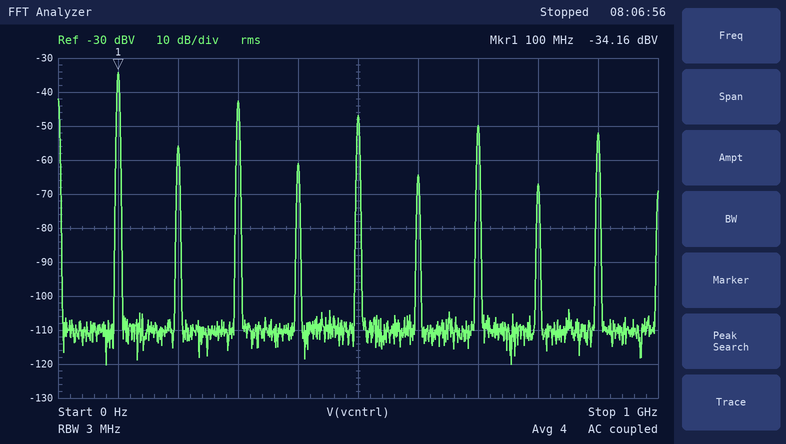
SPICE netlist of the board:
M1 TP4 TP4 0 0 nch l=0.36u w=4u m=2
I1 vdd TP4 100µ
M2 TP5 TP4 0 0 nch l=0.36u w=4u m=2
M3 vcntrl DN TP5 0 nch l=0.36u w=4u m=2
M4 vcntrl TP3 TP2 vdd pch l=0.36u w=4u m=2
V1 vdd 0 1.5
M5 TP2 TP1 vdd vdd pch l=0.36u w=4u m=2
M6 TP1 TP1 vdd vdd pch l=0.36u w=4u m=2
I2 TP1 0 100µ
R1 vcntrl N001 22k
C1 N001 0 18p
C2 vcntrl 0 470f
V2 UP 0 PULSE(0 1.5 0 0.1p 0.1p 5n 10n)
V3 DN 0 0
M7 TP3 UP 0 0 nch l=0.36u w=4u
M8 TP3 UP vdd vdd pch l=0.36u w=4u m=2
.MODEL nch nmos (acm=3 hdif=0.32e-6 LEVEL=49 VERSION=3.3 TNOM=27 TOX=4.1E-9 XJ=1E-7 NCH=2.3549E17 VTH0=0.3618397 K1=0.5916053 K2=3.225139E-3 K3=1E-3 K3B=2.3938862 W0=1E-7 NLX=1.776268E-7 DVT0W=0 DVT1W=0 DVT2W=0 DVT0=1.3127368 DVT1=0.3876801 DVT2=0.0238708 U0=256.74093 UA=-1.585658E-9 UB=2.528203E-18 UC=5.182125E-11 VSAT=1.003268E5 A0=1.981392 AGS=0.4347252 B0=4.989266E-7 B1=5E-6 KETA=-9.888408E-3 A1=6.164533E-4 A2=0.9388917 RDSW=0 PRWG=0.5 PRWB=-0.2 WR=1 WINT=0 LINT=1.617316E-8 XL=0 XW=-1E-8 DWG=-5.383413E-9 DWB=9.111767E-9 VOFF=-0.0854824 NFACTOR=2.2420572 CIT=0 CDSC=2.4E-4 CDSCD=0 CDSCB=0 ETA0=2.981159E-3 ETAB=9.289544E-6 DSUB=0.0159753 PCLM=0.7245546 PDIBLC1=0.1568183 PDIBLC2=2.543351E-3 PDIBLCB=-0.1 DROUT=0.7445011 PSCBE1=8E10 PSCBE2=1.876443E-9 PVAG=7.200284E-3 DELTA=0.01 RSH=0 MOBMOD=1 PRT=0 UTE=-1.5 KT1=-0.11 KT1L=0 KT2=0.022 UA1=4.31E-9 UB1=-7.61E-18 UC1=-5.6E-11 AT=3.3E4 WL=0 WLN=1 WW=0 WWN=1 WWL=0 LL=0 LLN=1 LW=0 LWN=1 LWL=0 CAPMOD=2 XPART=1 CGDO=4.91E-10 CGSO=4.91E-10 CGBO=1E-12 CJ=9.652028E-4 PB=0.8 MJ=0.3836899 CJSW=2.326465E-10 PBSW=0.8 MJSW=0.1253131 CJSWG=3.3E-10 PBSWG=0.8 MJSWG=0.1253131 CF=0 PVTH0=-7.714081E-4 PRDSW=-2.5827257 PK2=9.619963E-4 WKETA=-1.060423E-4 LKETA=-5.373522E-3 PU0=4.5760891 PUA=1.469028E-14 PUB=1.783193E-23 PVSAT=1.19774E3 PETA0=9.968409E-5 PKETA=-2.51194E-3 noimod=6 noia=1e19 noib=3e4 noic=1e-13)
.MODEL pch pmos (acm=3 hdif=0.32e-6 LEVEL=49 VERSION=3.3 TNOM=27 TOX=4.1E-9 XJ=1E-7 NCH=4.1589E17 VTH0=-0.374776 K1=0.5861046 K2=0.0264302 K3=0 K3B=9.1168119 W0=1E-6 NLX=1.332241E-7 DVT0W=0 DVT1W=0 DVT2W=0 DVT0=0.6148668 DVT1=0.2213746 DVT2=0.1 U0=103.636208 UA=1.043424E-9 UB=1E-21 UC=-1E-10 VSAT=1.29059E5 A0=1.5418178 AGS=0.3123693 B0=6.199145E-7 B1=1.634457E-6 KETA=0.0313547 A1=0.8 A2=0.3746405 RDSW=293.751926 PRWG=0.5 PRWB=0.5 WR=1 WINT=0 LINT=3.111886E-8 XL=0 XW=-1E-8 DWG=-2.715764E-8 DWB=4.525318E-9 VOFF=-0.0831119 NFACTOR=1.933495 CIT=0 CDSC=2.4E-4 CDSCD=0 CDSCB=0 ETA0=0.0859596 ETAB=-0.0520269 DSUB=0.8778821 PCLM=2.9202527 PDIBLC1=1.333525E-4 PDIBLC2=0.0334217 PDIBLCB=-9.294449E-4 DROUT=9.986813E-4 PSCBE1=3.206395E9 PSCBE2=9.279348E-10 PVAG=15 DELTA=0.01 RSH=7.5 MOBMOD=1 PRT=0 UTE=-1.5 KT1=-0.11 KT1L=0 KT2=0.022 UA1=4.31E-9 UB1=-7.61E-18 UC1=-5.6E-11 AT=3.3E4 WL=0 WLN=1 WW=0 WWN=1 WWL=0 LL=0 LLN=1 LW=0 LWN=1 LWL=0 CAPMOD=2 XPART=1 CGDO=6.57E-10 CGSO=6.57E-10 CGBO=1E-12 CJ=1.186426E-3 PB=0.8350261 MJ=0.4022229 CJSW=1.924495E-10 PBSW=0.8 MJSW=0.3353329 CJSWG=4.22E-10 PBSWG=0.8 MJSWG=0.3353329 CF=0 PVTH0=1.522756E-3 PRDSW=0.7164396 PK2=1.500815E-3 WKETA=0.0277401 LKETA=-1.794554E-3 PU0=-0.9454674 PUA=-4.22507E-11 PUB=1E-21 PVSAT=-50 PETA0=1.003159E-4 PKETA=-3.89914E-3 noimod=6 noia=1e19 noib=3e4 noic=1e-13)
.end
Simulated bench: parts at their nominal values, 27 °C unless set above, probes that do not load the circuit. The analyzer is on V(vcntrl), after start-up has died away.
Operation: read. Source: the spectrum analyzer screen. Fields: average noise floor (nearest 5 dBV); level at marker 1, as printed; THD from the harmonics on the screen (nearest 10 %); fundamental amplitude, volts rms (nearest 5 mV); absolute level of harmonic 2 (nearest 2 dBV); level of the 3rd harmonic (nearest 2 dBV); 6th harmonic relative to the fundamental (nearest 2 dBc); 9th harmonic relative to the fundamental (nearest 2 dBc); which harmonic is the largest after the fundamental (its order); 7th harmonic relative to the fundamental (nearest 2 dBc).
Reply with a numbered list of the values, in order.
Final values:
1. -110 dBV
2. -34.16 dBV
3. 50 %
4. 20 mV
5. -56 dBV
6. -42 dBV
7. -30 dBc
8. -18 dBc
9. 3
10. -16 dBc
